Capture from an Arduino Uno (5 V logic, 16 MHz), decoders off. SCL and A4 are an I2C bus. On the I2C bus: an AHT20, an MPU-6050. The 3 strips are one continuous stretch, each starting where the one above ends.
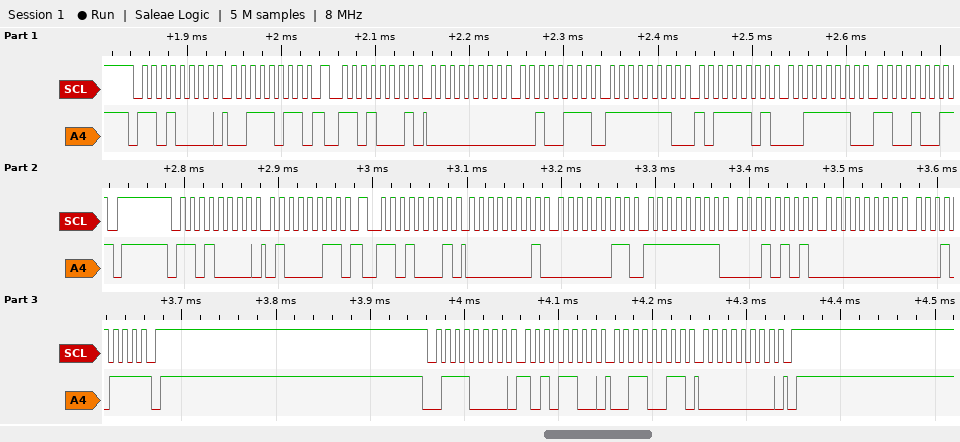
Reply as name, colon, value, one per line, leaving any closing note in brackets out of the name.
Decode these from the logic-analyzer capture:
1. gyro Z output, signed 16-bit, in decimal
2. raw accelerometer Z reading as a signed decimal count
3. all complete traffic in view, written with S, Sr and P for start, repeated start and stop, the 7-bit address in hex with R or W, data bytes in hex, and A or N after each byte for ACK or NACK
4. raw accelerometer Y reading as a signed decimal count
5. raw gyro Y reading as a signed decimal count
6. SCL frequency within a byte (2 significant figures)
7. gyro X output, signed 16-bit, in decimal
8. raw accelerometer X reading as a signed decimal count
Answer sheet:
gyro Z output, signed 16-bit, in decimal: 23
raw accelerometer Z reading as a signed decimal count: 16073
all complete traffic in view, written with S, Sr and P for start, repeated start and stop, the 7-bit address in hex with R or W, data bytes in hex, and A or N after each byte for ACK or NACK: S 68W A 3B A Sr 68R A 00 A 27 A FE A BD A 3E A C9 N P S 68W A 43 A Sr 68R A 01 A 03 A FF A 15 A 00 A 17 N P S 38W A AC A 33 A 00 A P
raw accelerometer Y reading as a signed decimal count: -323
raw gyro Y reading as a signed decimal count: -235
SCL frequency within a byte: 100 kHz
gyro X output, signed 16-bit, in decimal: 259
raw accelerometer X reading as a signed decimal count: 39
